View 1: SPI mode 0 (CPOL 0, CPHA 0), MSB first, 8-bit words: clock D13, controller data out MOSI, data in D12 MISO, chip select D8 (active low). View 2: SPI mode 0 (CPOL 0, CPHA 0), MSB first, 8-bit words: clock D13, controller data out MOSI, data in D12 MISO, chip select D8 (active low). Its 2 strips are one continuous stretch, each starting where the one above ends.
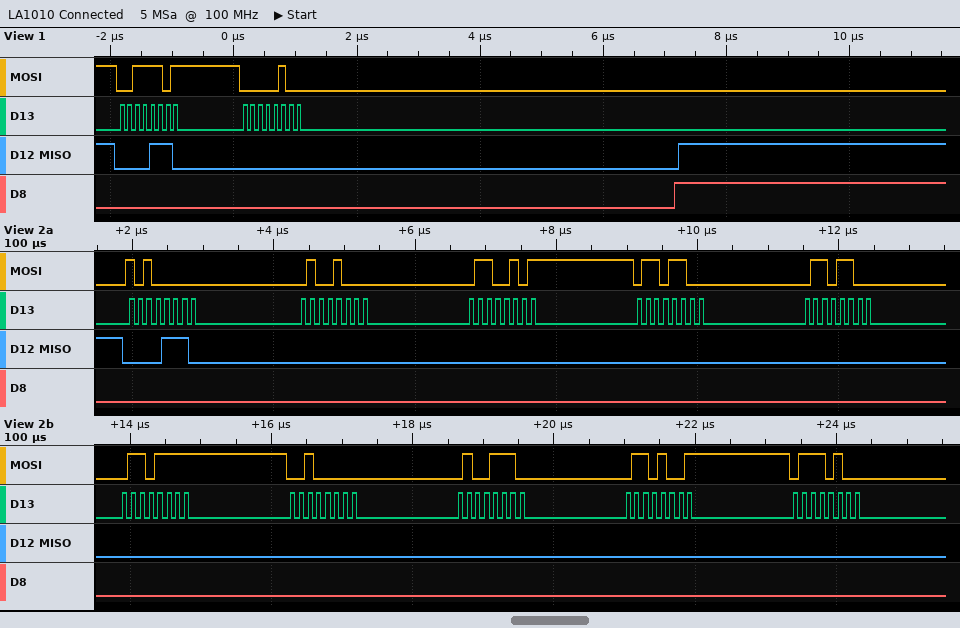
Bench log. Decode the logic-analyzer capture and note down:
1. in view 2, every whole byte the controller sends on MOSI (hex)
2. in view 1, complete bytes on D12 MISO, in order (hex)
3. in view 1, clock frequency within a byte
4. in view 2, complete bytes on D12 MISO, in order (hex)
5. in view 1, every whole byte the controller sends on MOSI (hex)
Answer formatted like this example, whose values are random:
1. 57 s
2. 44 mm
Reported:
1. A0 48 65 6C 6C 6F 20 4E 69 74
2. 0x0E 0x00
3. 8 MHz
4. 0E 00 00 00 00 00 00 00 00 00
5. 0x3D 0x04
